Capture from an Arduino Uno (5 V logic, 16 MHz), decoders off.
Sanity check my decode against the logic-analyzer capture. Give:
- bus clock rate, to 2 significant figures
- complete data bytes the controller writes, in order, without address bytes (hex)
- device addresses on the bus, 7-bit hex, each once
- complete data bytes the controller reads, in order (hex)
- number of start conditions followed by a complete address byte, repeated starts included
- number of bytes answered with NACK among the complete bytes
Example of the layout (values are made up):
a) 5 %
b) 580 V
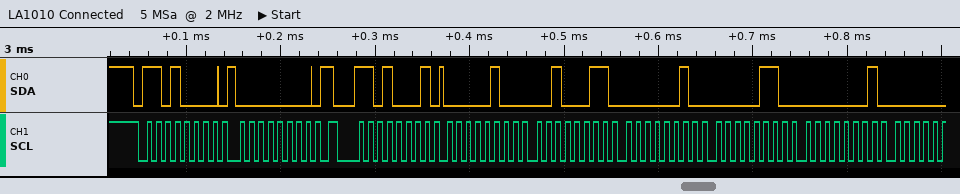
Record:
a) 100 kHz
b) 00
c) 0x68
d) 04 23 02 06 01
e) 2
f) 0
